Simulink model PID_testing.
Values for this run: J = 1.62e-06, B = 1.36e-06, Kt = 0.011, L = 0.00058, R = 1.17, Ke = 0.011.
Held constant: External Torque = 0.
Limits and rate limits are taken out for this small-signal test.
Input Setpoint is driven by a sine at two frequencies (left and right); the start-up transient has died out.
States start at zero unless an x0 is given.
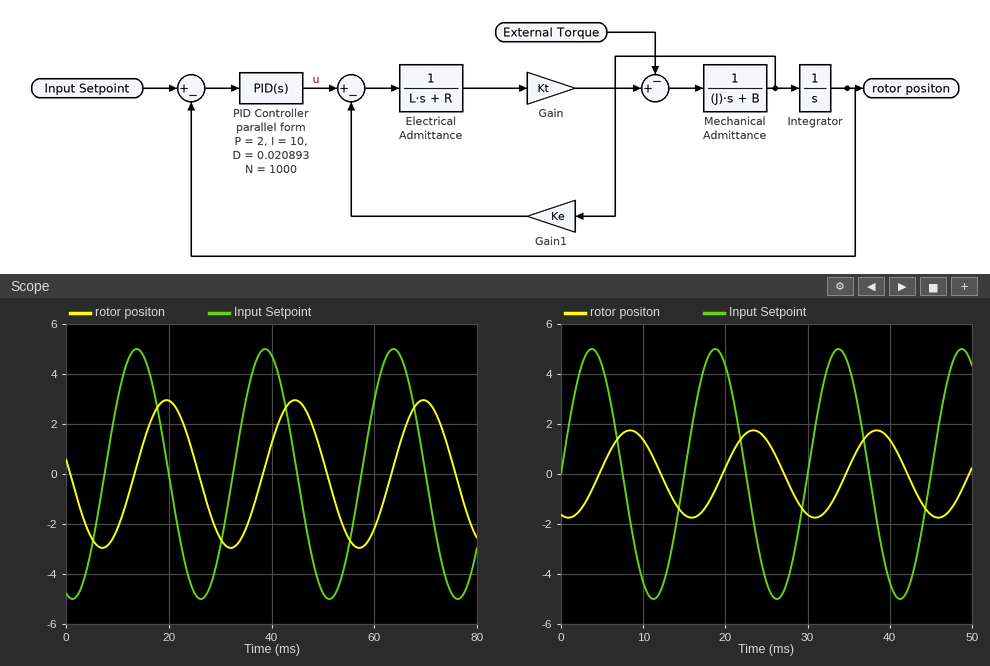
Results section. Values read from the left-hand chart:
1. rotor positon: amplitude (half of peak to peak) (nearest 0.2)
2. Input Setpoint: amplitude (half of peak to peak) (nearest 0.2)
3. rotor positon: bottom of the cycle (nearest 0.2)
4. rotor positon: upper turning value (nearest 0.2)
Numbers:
3.0
5.0
-3.0
3.0
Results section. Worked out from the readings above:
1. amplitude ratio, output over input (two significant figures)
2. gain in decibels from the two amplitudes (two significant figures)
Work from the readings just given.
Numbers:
0.60
-4.4 dB
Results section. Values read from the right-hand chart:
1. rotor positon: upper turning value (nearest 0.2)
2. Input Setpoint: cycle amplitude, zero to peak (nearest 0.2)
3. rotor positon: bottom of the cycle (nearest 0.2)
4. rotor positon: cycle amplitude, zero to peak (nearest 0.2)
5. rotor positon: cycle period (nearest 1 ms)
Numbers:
1.8
5.0
-1.8
1.8
15 ms
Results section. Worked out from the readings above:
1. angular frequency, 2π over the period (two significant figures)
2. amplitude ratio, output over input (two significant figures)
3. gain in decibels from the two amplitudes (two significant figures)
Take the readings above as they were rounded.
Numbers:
0.42 rad/ms
0.36
-8.9 dB
